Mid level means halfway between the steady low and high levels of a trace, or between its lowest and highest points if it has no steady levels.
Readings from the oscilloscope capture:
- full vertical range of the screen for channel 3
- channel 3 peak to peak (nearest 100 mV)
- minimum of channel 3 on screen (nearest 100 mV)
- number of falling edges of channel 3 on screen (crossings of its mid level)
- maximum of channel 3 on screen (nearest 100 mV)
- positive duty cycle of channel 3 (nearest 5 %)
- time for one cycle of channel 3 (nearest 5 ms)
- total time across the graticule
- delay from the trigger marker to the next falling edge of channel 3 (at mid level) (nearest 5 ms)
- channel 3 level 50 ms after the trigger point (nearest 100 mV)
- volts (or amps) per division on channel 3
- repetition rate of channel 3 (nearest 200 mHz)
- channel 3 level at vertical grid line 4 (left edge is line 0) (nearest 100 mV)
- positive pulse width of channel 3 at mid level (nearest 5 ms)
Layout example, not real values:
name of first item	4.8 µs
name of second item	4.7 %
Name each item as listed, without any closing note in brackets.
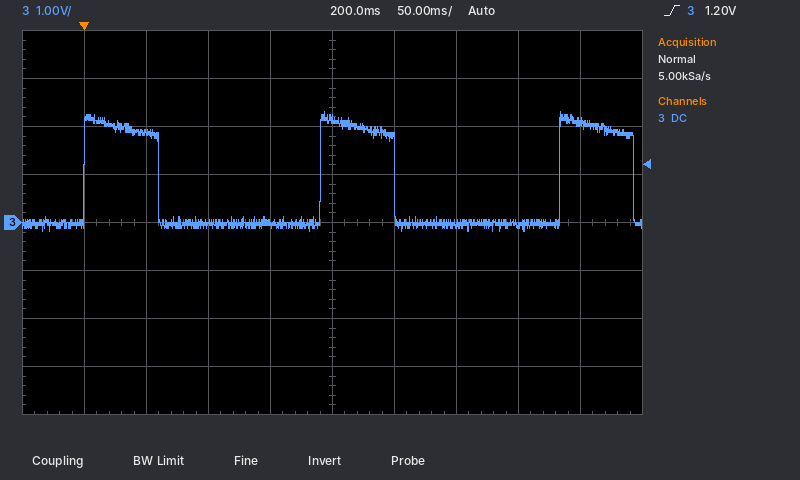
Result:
full vertical range of the screen for channel 3	8 V
channel 3 peak to peak	2.5 V
minimum of channel 3 on screen	-200 mV
number of falling edges of channel 3 on screen	3
maximum of channel 3 on screen	2.3 V
positive duty cycle of channel 3	30 %
time for one cycle of channel 3	190 ms
total time across the graticule	500 ms
delay from the trigger marker to the next falling edge of channel 3 (at mid level)	60 ms
channel 3 level 50 ms after the trigger point	1.9 V
volts (or amps) per division on channel 3	1 V
repetition rate of channel 3	5.2 Hz
channel 3 level at vertical grid line 4 (left edge is line 0)	0.0 V
positive pulse width of channel 3 at mid level	60 ms
